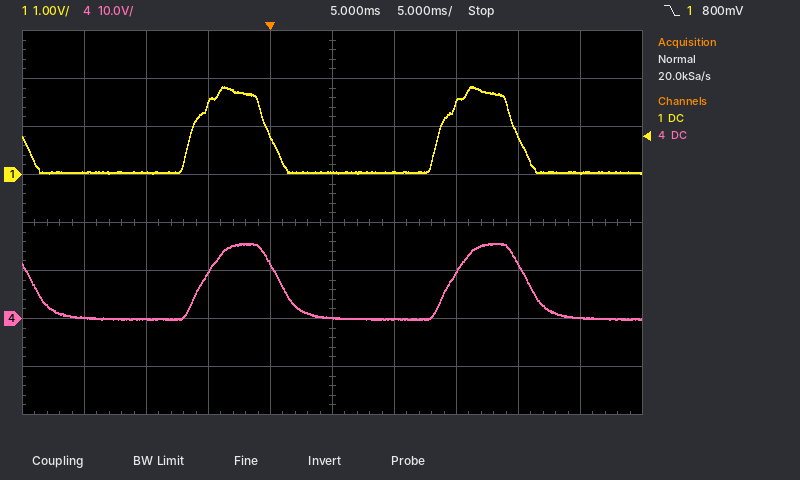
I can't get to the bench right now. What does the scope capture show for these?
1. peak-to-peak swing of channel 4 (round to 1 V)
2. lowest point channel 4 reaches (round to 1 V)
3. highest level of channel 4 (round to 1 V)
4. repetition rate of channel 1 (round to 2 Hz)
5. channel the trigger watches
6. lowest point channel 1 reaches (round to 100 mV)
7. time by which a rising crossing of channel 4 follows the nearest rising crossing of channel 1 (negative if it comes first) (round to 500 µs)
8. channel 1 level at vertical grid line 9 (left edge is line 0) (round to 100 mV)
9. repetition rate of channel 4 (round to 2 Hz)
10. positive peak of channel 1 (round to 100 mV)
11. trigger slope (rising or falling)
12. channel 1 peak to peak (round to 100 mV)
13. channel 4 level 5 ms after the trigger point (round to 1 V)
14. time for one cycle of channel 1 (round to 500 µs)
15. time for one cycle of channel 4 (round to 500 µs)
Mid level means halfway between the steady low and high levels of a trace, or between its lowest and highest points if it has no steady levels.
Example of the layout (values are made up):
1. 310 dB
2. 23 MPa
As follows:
1. 16 V
2. 0 V
3. 16 V
4. 50 Hz
5. channel 1
6. 0.0 V
7. +1.0 ms
8. 0.0 V
9. 50 Hz
10. 1.8 V
11. falling
12. 1.8 V
13. 0 V
14. 20.0 ms
15. 20.0 ms
